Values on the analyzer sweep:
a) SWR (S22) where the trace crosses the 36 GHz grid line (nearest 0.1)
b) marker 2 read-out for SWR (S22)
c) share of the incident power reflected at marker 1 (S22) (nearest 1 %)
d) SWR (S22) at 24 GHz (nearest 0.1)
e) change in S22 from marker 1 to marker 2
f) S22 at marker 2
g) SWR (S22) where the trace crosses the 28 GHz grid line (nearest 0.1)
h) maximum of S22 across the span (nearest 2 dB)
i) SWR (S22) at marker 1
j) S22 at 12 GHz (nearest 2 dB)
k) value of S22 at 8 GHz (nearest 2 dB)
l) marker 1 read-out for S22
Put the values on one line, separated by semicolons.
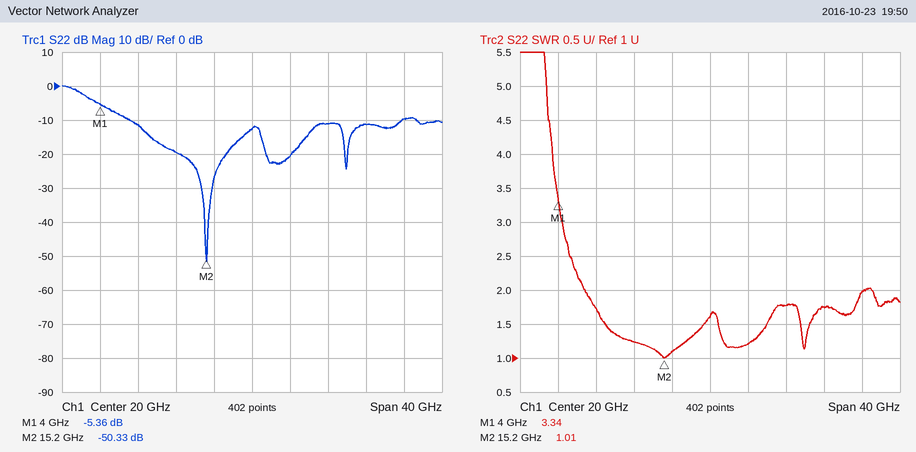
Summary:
2.0; 1.01; 29 %; 1.2; -44.97 dB; -50.33 dB; 1.8; 0 dB; 3.34; -20 dB; -12 dB; -5.36 dB
